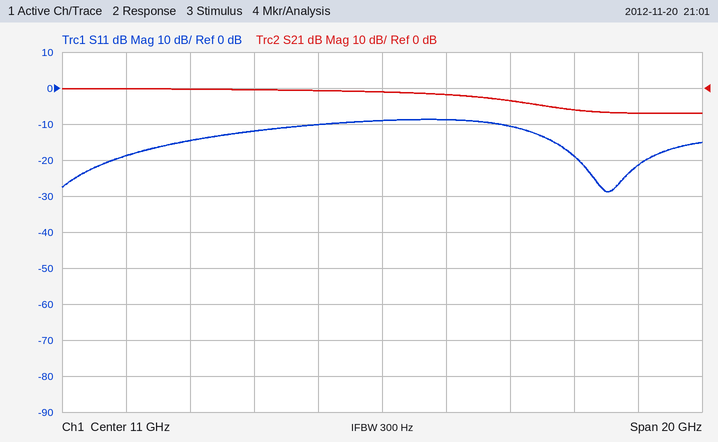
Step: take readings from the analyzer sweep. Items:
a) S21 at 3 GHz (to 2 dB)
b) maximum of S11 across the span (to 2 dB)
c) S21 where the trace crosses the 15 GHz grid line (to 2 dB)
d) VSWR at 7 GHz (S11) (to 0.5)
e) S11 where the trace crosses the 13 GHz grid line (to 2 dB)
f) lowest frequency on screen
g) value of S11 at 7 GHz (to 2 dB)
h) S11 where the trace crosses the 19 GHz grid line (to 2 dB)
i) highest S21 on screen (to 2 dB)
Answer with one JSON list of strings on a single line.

["0 dB", "-8 dB", "-4 dB", "1.5", "-8 dB", "1 GHz", "-12 dB", "-22 dB", "0 dB"]
